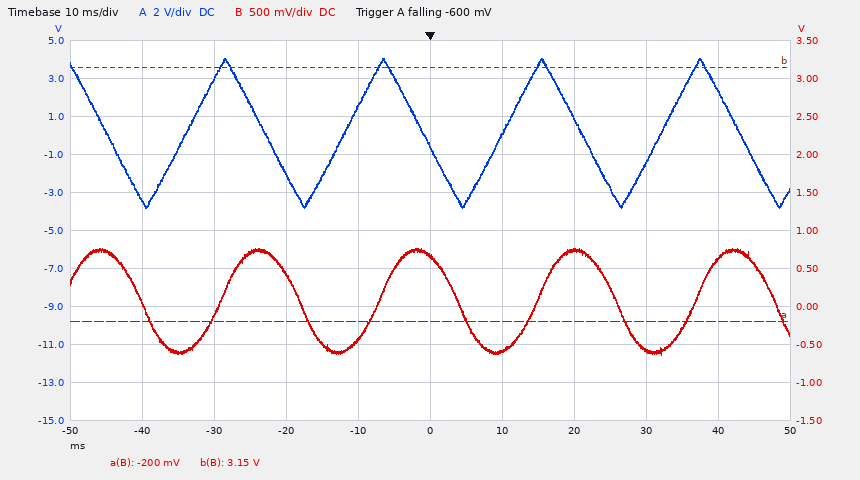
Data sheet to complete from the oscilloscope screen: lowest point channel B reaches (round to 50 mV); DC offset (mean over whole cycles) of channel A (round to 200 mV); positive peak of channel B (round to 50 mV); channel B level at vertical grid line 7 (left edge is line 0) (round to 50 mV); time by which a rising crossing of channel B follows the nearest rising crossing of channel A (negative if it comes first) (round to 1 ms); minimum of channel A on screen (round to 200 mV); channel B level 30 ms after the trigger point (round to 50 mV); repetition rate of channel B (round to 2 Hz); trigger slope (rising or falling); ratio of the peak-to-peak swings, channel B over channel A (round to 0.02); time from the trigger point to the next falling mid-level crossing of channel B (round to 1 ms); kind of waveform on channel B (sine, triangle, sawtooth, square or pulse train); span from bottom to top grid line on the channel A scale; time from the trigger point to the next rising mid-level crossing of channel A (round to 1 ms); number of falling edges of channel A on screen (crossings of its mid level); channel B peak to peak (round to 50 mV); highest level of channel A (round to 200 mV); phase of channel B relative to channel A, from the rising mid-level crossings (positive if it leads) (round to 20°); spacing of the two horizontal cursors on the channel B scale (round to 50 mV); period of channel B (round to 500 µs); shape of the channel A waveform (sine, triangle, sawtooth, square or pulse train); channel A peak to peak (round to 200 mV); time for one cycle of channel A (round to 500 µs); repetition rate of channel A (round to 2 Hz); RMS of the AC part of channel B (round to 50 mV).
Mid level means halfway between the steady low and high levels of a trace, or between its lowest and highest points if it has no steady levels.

-650 mV
200 mV
750 mV
750 mV
+5 ms
-3.8 V
-550 mV
46 Hz
falling
0.18
4 ms
sine
20 V
10 ms
5
1.40 V
4.0 V
-80°
3.35 V
22.0 ms
triangle
7.8 V
22.0 ms
46 Hz
500 mV
